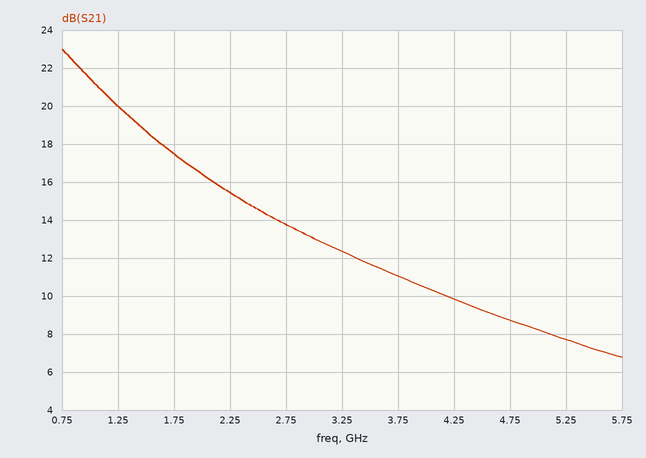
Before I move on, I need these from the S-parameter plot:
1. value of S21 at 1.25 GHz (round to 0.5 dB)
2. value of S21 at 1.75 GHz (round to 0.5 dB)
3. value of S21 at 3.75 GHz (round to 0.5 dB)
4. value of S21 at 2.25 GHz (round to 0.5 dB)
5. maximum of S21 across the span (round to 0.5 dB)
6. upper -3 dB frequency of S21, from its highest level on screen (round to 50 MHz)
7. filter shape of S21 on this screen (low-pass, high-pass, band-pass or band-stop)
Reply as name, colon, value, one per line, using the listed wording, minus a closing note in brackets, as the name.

value of S21 at 1.25 GHz: 20.0 dB
value of S21 at 1.75 GHz: 17.5 dB
value of S21 at 3.75 GHz: 11.0 dB
value of S21 at 2.25 GHz: 15.5 dB
maximum of S21 across the span: 23.0 dB
upper -3 dB frequency of S21, from its highest level on screen: 1.25 GHz
filter shape of S21 on this screen: low-pass
